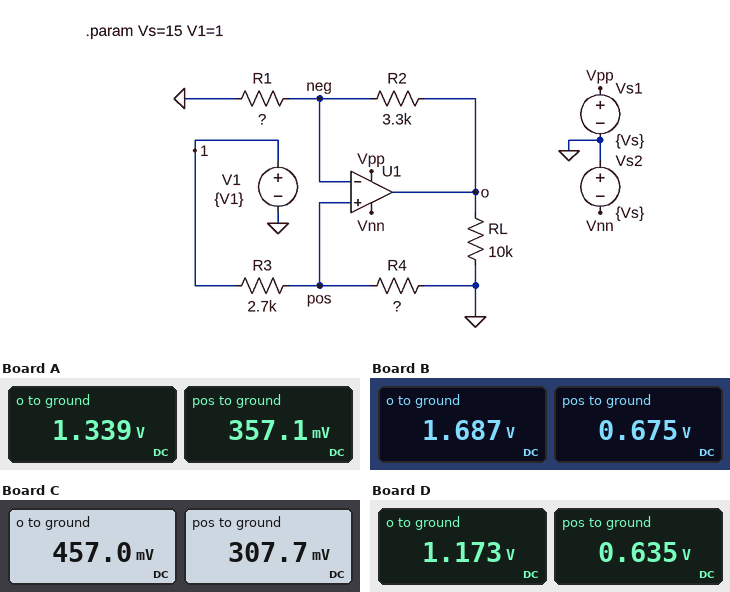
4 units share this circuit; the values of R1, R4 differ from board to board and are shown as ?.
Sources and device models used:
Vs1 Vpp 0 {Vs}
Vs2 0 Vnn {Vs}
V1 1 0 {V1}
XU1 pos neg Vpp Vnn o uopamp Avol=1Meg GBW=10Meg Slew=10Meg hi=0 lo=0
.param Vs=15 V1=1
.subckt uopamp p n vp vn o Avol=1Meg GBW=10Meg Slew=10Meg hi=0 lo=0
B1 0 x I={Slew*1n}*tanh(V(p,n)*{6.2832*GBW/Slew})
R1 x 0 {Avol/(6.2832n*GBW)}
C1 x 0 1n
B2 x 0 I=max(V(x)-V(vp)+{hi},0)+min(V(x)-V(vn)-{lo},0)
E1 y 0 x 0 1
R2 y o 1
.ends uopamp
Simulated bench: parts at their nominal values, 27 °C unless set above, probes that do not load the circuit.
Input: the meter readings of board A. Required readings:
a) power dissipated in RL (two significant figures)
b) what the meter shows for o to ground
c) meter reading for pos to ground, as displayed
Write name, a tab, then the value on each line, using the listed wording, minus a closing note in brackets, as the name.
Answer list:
power dissipated in RL	180 µW
what the meter shows for o to ground	1.339 V
meter reading for pos to ground, as displayed	357.1 mV
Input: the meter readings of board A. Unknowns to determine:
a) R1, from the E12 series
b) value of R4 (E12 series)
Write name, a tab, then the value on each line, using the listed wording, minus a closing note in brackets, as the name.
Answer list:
R1, from the E12 series	1.2 kΩ
value of R4	1.5 kΩ
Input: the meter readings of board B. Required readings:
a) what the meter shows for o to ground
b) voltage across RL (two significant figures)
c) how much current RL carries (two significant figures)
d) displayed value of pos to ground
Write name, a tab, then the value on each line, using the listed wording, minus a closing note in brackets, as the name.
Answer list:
what the meter shows for o to ground	1.687 V
voltage across RL	1.7 V
how much current RL carries	170 µA
displayed value of pos to ground	0.675 V
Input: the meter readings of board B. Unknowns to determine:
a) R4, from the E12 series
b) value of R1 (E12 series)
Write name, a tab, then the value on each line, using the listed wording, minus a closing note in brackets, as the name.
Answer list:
R4, from the E12 series	5.6 kΩ
value of R1	2.2 kΩ
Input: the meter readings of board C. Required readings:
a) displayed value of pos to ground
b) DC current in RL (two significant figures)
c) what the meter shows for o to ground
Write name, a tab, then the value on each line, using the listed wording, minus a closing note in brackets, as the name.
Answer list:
displayed value of pos to ground	307.7 mV
DC current in RL	46 µA
what the meter shows for o to ground	457.0 mV
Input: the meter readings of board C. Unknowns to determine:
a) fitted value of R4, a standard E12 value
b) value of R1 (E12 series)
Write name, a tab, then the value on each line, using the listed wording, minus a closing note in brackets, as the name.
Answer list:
fitted value of R4, a standard E12 value	1.2 kΩ
value of R1	6.8 kΩ
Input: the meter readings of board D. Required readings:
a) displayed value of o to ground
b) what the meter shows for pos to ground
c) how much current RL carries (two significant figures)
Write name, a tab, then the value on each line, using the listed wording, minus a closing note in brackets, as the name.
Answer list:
displayed value of o to ground	1.173 V
what the meter shows for pos to ground	0.635 V
how much current RL carries	120 µA
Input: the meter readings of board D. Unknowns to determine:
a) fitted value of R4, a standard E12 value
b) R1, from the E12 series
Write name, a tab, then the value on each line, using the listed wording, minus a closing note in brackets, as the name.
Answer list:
fitted value of R4, a standard E12 value	4.7 kΩ
R1, from the E12 series	3.9 kΩ
